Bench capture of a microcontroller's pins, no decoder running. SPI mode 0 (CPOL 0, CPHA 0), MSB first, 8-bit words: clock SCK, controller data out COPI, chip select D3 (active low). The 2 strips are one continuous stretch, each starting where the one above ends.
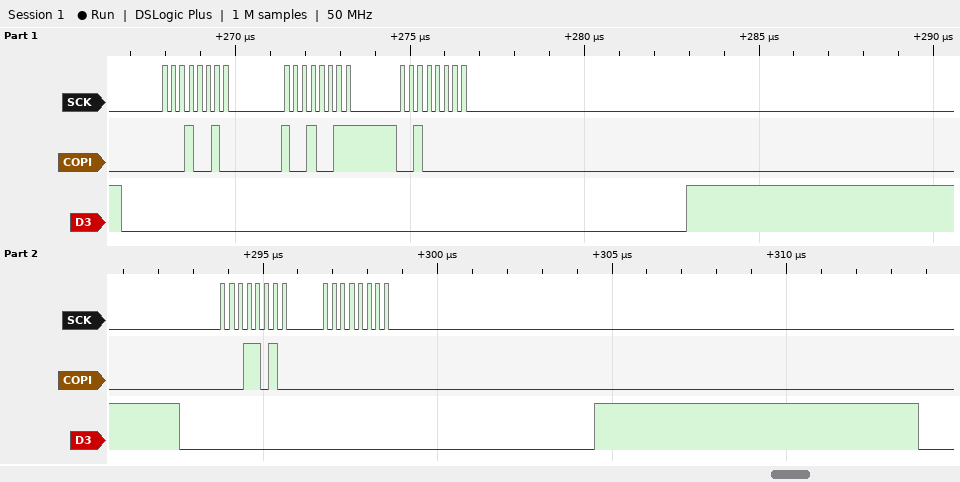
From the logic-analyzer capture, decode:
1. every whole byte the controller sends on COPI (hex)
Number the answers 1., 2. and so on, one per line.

1. 12 93 20 1A 00
